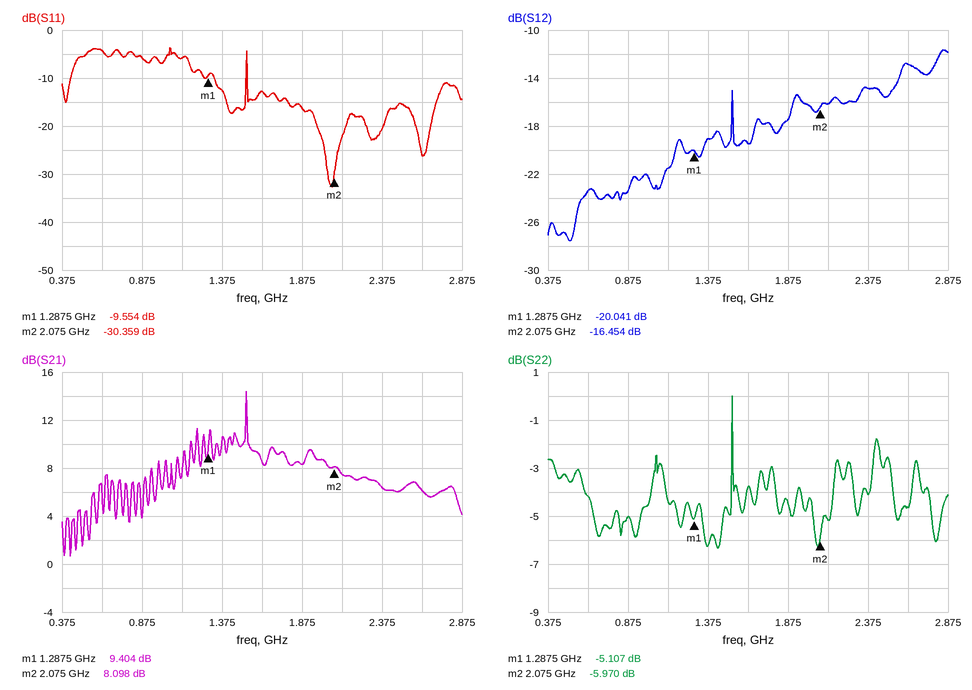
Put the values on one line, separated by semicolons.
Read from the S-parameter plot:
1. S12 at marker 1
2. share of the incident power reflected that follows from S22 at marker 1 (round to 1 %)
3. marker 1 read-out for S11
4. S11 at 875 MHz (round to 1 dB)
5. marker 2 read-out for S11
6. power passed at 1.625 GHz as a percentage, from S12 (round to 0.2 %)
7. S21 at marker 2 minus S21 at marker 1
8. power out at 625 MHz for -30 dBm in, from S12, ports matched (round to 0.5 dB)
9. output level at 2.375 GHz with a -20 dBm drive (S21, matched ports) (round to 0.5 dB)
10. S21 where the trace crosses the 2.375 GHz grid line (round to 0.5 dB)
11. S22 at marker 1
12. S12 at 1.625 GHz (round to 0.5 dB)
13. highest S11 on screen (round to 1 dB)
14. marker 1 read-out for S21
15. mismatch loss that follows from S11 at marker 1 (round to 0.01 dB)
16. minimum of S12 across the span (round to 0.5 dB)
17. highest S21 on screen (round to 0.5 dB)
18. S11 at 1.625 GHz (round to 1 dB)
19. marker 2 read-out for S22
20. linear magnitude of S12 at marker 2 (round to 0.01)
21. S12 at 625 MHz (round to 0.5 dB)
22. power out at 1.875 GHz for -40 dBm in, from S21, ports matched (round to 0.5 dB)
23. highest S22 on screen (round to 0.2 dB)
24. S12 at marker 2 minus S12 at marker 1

-20.041 dB; 31 %; -9.554 dB; -6 dB; -30.359 dB; 1.2 %; -1.306 dB; -53.5 dBm; -13.5 dBm; 6.5 dB; -5.107 dB; -19.5 dB; -4 dB; 9.404 dB; 0.51 dB; -27.5 dB; 14.5 dB; -13 dB; -5.970 dB; 0.15; -23.5 dB; -31.5 dBm; 0.0 dB; 3.587 dB
